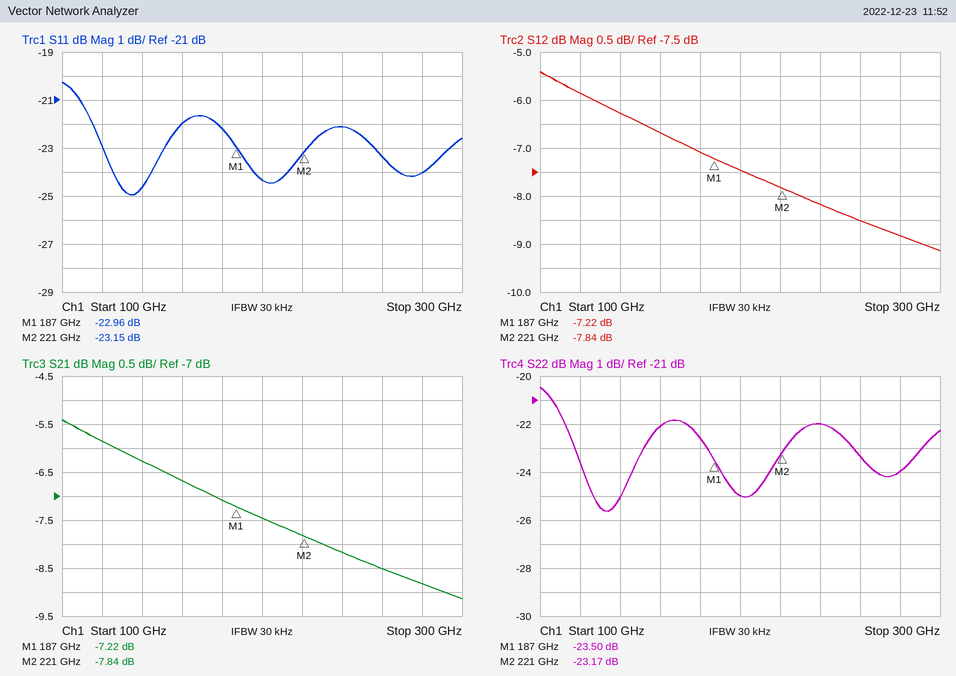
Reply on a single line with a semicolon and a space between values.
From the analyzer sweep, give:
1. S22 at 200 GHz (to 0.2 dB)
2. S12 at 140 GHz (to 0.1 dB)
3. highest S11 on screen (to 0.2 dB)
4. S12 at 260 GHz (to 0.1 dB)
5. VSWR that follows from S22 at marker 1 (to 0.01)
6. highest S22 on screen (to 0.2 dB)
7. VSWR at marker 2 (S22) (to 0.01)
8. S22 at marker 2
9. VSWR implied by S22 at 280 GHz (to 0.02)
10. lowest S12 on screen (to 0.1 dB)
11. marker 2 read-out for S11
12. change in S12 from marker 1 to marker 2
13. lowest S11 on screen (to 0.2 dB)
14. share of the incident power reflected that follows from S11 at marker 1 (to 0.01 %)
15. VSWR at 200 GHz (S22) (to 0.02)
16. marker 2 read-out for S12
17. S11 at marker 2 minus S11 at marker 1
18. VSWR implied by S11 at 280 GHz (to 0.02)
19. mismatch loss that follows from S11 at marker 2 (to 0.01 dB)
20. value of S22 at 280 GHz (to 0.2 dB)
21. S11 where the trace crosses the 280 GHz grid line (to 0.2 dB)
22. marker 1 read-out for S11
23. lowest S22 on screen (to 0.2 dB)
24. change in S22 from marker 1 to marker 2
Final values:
-25.0 dB; -6.3 dB; -20.2 dB; -8.5 dB; 1.14; -20.4 dB; 1.15; -23.17 dB; 1.14; -9.1 dB; -23.15 dB; -0.62 dB; -25.0 dB; 0.51 %; 1.12; -7.84 dB; -0.19 dB; 1.14; 0.02 dB; -24.0 dB; -24.0 dB; -22.96 dB; -25.6 dB; 0.33 dB
